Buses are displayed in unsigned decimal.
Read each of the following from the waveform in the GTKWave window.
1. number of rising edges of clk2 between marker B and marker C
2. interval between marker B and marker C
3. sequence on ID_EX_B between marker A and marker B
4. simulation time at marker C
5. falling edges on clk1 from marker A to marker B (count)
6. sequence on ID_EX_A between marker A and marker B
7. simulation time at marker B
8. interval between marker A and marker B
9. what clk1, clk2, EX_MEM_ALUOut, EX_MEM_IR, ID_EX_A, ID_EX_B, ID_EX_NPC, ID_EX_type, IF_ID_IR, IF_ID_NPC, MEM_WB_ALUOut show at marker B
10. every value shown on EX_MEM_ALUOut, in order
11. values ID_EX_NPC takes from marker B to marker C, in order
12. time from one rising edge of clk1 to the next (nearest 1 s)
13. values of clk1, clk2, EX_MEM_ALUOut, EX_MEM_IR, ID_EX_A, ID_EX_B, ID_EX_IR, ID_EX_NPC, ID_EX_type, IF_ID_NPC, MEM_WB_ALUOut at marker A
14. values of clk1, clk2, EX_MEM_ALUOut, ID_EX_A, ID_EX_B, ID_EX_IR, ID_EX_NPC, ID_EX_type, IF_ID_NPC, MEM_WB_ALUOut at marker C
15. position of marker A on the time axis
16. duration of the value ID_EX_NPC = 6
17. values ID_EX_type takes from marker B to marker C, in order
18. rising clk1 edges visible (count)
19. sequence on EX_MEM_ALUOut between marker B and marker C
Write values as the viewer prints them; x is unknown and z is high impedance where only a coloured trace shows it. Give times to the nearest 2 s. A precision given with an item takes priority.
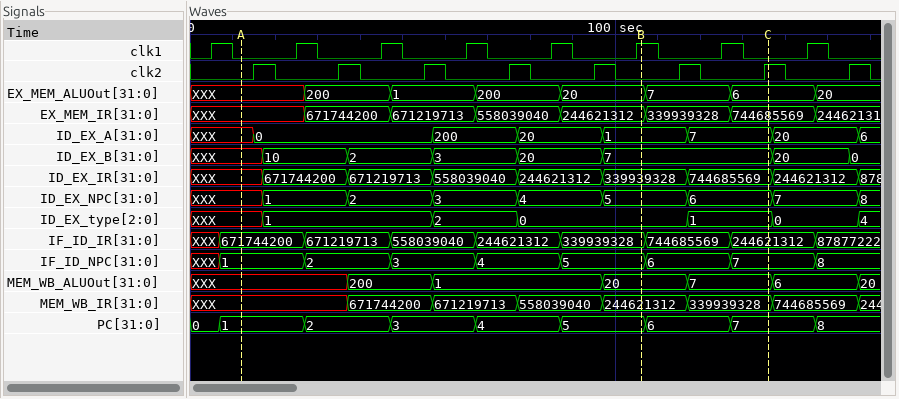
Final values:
2
30 s
XXX, 10, 2, 3, 20, 7
136 s
4
XXX, 0, 200, 20, 1
106 s
94 s
clk1=1, clk2=0, EX_MEM_ALUOut=20, EX_MEM_IR=244621312, ID_EX_A=1, ID_EX_B=7, ID_EX_NPC=5, ID_EX_type=0, IF_ID_IR=339939328, IF_ID_NPC=5, MEM_WB_ALUOut=20
XXX, 200, 1, 200, 20, 7, 6, 20
5, 6
20 s
clk1=0, clk2=0, EX_MEM_ALUOut=XXX, EX_MEM_IR=XXX, ID_EX_A=XXX, ID_EX_B=XXX, ID_EX_IR=XXX, ID_EX_NPC=XXX, ID_EX_type=XXX, IF_ID_NPC=1, MEM_WB_ALUOut=XXX
clk1=0, clk2=1, EX_MEM_ALUOut=6, ID_EX_A=7, ID_EX_B=7, ID_EX_IR=744685569, ID_EX_NPC=6, ID_EX_type=1, IF_ID_NPC=7, MEM_WB_ALUOut=7
12 s
20 s
0, 1
8
20, 7, 6
